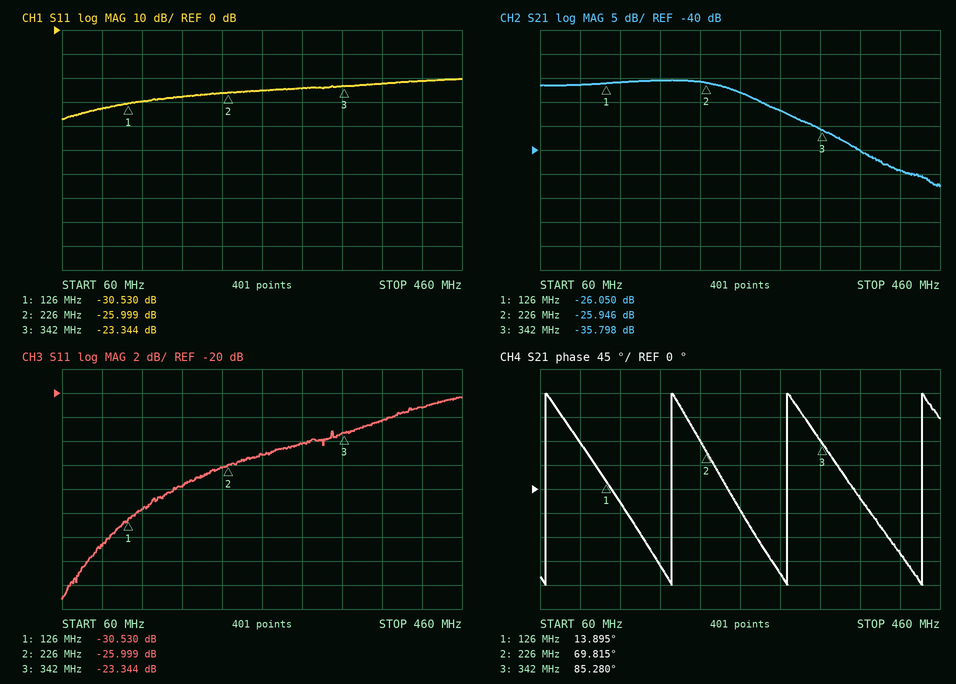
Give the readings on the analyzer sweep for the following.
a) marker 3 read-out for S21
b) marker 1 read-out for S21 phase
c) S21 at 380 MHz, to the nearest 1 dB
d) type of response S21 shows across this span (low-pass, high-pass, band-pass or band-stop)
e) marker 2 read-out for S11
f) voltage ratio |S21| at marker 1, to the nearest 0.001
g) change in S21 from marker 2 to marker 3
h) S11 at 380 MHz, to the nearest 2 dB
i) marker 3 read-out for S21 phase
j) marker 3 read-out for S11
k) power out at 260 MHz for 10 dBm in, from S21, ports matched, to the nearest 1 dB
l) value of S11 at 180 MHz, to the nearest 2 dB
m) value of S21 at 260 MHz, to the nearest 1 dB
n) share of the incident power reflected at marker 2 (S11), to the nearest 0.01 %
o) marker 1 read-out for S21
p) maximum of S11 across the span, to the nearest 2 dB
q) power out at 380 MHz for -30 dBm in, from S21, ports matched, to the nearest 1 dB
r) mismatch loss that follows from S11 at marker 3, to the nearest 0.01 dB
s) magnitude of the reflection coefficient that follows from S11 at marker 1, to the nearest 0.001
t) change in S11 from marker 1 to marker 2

-35.798 dB
13.895°
-40 dB
low-pass
-25.999 dB
0.050
-9.852 dB
-22 dB
85.280°
-23.344 dB
-18 dBm
-28 dB
-28 dB
0.25 %
-26.050 dB
-20 dB
-70 dBm
0.02 dB
0.030
4.531 dB
